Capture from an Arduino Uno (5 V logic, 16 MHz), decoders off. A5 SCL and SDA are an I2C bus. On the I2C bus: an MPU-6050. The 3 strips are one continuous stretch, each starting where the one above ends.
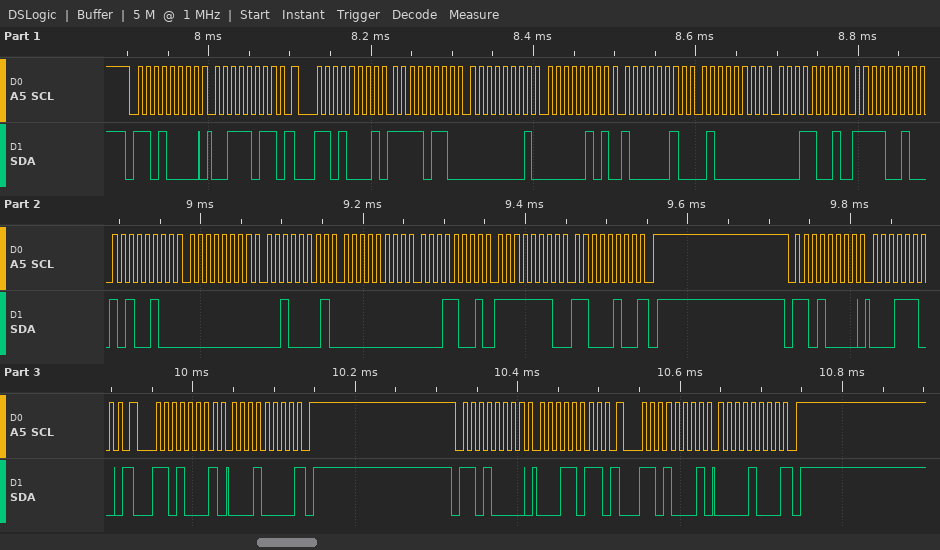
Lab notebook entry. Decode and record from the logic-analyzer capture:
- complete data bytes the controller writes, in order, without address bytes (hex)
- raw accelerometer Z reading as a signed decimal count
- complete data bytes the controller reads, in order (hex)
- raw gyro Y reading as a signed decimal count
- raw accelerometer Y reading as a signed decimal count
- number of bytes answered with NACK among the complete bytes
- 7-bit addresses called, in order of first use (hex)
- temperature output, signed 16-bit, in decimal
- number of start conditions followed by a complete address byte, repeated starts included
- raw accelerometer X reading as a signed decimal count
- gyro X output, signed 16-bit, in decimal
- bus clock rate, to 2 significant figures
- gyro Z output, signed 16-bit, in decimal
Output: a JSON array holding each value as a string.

["3B 1C 1B", "16409", "F6 01 05 82 40 19 F2 A4 00 21 00 19 FE C4 10 08", "25", "1410", "3", "0x68", "-3420", "6", "-2559", "33", "100 kHz", "-316"]
